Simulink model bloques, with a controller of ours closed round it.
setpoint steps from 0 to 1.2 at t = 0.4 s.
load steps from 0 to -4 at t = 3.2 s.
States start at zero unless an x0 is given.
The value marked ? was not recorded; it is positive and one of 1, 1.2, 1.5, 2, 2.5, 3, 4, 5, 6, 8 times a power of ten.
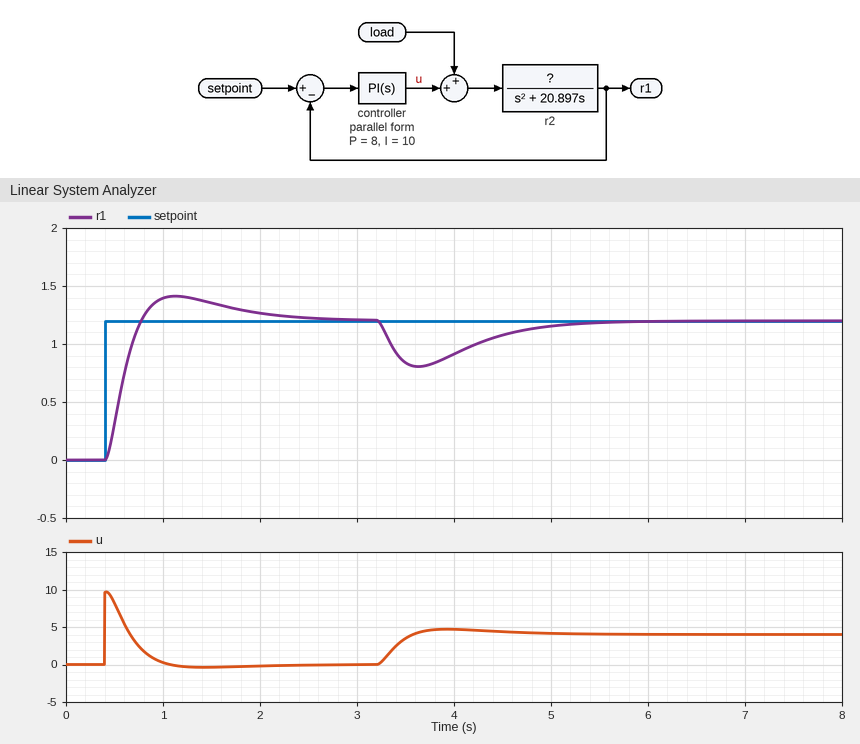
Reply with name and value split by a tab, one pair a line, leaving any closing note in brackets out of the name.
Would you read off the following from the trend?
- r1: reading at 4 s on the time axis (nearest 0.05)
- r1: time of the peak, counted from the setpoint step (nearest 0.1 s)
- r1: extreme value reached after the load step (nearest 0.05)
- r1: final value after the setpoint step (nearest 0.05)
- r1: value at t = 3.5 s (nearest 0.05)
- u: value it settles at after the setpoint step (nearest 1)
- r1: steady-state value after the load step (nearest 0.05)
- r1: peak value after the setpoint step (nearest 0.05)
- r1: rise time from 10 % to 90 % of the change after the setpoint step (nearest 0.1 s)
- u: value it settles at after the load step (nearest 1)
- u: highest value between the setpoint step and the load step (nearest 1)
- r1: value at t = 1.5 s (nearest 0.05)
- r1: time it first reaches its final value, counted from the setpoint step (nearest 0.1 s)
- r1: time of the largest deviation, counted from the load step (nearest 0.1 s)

r1: reading at 4 s on the time axis	0.90
r1: time of the peak, counted from the setpoint step	0.7 s
r1: extreme value reached after the load step	0.80
r1: final value after the setpoint step	1.20
r1: value at t = 3.5 s	0.85
u: value it settles at after the setpoint step	0
r1: steady-state value after the load step	1.20
r1: peak value after the setpoint step	1.40
r1: rise time from 10 % to 90 % of the change after the setpoint step	0.3 s
u: value it settles at after the load step	4
u: highest value between the setpoint step and the load step	10
r1: value at t = 1.5 s	1.35
r1: time it first reaches its final value, counted from the setpoint step	0.4 s
r1: time of the largest deviation, counted from the load step	0.4 s
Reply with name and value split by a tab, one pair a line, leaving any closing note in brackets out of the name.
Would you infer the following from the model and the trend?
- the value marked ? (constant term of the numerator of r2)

the value marked ?	12
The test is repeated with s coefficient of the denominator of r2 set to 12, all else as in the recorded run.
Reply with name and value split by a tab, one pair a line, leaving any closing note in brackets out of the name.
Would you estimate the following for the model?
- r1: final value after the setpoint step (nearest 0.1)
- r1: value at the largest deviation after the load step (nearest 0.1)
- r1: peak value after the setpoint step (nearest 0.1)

r1: final value after the setpoint step	1.2
r1: value at the largest deviation after the load step	0.7
r1: peak value after the setpoint step	1.5
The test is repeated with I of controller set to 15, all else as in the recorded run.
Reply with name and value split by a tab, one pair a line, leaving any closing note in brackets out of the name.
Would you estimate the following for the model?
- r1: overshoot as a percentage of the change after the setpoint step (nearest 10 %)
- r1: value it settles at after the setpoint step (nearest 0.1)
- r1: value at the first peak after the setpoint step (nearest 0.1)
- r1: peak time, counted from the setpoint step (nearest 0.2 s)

r1: overshoot as a percentage of the change after the setpoint step	20 %
r1: value it settles at after the setpoint step	1.2
r1: value at the first peak after the setpoint step	1.5
r1: peak time, counted from the setpoint step	0.6 s
